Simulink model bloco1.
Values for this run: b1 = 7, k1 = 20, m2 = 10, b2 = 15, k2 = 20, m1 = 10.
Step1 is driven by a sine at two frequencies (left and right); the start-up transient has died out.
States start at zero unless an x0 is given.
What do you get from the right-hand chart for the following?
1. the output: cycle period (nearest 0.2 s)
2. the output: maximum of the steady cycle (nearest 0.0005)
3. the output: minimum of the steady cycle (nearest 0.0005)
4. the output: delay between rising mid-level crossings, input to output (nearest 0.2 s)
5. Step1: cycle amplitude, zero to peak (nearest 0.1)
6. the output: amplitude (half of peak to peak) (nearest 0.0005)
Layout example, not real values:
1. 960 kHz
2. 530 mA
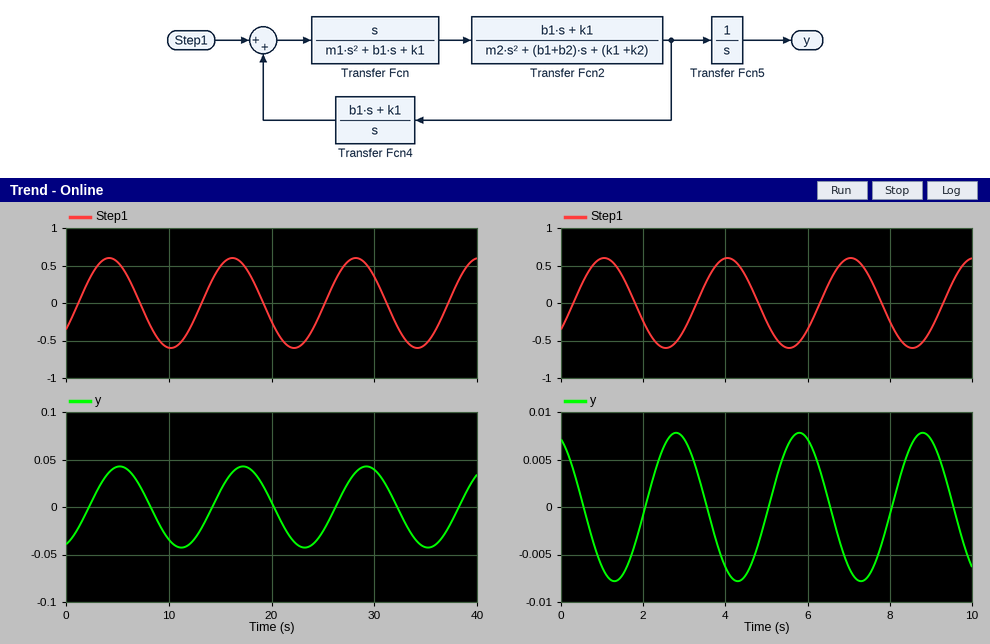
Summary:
1. 3.0 s
2. 0.0080
3. -0.0080
4. 1.8 s
5. 0.6
6. 0.0080
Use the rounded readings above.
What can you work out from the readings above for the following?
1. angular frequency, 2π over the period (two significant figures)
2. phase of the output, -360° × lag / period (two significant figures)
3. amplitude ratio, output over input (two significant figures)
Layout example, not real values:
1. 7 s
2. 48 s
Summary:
1. 2.1 rad/s
2. -220°
3. 0.013
